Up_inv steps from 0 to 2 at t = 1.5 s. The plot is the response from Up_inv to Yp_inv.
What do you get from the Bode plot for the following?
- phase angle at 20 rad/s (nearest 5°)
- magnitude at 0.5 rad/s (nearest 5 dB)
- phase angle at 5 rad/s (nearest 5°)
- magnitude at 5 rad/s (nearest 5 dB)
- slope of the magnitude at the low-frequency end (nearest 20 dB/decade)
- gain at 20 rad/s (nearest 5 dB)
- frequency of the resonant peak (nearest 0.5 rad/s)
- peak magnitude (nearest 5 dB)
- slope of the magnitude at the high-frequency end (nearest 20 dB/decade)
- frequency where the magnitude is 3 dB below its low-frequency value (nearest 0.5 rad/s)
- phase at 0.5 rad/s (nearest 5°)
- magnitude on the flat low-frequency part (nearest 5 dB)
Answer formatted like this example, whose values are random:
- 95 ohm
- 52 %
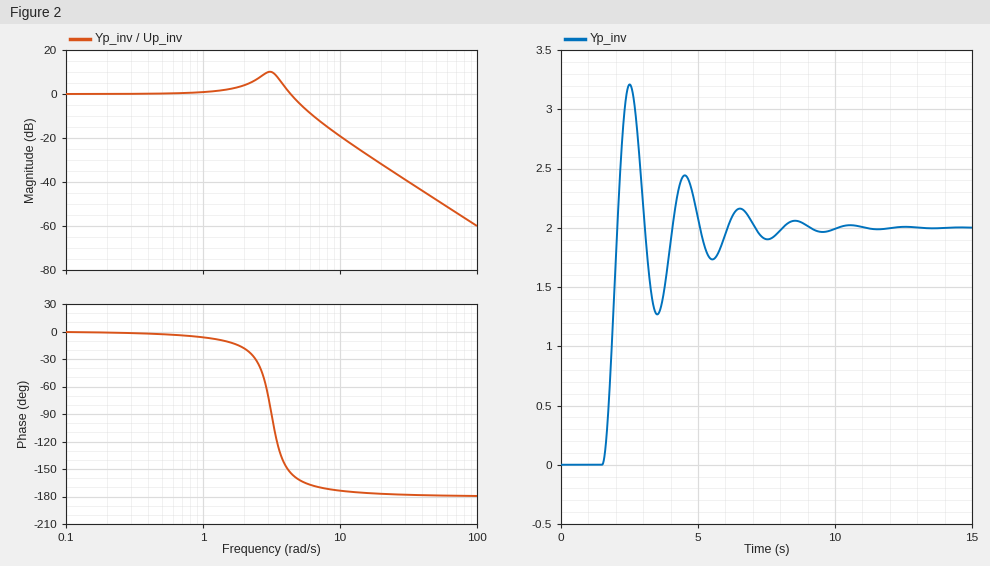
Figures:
- -175°
- 0 dB
- -160°
- -5 dB
- 0 dB/decade
- -30 dB
- 3.0 rad/s
- 10 dB
- -40 dB/decade
- 5.0 rad/s
- -5°
- 0 dB
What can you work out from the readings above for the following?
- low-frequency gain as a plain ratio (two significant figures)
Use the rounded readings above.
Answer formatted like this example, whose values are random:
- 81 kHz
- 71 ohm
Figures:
- 1.0
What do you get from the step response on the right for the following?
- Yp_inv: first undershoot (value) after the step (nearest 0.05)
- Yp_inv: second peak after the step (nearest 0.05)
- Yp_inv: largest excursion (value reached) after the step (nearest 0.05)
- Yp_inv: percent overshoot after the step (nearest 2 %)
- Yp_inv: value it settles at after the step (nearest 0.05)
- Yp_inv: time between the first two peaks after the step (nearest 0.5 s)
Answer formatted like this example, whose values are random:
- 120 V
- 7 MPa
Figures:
- 1.25
- 2.45
- 3.20
- 60 %
- 2.00
- 2.0 s
